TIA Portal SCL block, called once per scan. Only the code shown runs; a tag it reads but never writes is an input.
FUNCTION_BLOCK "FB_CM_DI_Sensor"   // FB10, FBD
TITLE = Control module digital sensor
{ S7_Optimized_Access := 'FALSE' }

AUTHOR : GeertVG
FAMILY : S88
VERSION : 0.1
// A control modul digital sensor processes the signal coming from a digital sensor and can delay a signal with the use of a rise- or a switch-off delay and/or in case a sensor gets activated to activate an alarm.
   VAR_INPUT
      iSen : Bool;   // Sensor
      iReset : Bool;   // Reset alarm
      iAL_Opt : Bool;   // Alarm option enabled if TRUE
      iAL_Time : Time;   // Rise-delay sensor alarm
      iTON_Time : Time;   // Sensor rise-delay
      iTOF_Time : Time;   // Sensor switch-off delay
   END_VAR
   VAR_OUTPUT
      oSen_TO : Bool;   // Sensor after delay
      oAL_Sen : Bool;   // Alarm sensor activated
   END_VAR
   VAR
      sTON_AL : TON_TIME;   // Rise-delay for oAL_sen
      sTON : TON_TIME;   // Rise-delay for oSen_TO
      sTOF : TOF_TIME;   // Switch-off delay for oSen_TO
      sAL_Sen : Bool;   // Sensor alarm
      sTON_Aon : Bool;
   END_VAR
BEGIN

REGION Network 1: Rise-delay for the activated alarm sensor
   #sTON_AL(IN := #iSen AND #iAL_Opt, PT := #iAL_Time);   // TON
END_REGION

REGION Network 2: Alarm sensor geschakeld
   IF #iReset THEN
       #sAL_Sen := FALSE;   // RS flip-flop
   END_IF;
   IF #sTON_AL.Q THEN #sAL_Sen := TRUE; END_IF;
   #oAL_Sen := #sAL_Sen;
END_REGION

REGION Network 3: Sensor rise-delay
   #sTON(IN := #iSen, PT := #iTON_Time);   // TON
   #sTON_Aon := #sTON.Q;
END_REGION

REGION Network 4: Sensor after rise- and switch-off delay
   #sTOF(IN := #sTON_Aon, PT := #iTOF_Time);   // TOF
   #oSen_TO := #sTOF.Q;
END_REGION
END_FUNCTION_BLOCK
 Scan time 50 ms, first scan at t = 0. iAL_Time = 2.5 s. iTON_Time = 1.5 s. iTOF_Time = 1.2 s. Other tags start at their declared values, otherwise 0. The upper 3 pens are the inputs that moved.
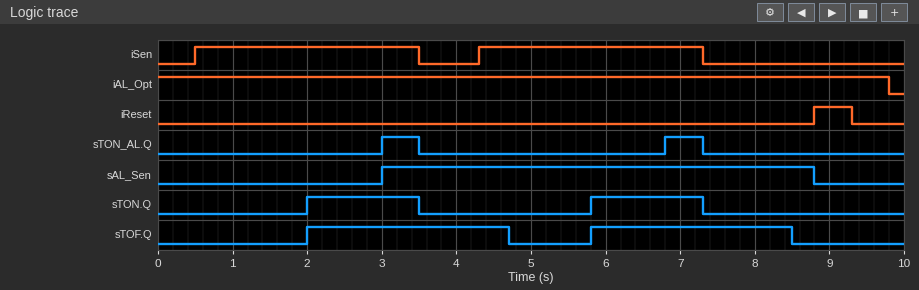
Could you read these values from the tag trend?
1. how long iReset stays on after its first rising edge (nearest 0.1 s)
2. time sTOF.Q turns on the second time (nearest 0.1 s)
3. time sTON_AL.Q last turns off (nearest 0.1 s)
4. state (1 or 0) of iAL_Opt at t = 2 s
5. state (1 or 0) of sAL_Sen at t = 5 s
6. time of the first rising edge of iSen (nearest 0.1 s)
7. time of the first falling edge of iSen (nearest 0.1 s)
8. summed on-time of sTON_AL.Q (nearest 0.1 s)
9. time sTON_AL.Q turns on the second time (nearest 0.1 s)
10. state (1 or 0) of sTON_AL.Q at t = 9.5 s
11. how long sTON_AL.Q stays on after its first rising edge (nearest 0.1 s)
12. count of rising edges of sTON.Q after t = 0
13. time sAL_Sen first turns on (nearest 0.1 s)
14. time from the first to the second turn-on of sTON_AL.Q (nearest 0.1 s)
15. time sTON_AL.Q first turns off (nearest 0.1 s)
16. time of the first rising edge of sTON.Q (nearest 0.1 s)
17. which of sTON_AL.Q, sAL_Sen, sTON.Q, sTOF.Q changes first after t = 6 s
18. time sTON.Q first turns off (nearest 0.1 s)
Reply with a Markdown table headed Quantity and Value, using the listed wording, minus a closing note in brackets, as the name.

| Quantity | Value |
|---|---|
| how long iReset stays on after its first rising edge | 0.5 s |
| time sTOF.Q turns on the second time | 5.8 s |
| time sTON_AL.Q last turns off | 7.3 s |
| state (1 or 0) of iAL_Opt at t = 2 s | 1 |
| state (1 or 0) of sAL_Sen at t = 5 s | 1 |
| time of the first rising edge of iSen | 0.5 s |
| time of the first falling edge of iSen | 3.5 s |
| summed on-time of sTON_AL.Q | 1.0 s |
| time sTON_AL.Q turns on the second time | 6.8 s |
| state (1 or 0) of sTON_AL.Q at t = 9.5 s | 0 |
| how long sTON_AL.Q stays on after its first rising edge | 0.5 s |
| count of rising edges of sTON.Q after t = 0 | 2 |
| time sAL_Sen first turns on | 3.0 s |
| time from the first to the second turn-on of sTON_AL.Q | 3.8 s |
| time sTON_AL.Q first turns off | 3.5 s |
| time of the first rising edge of sTON.Q | 2.0 s |
| which of sTON_AL.Q, sAL_Sen, sTON.Q, sTOF.Q changes first after t = 6 s | sTON_AL.Q |
| time sTON.Q first turns off | 3.5 s |
